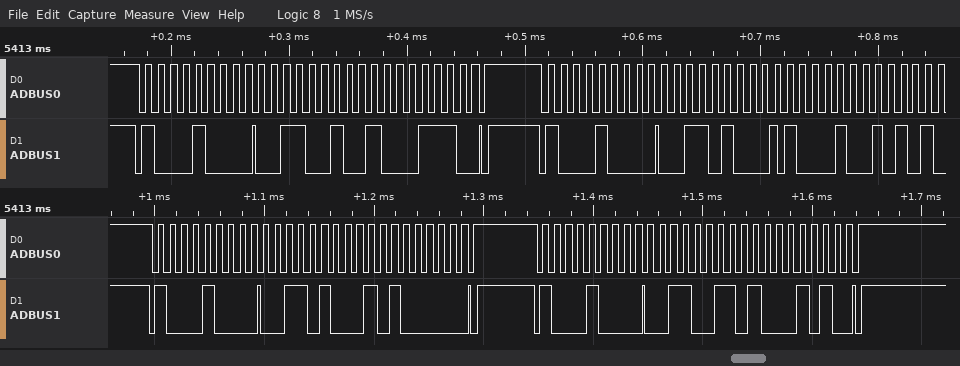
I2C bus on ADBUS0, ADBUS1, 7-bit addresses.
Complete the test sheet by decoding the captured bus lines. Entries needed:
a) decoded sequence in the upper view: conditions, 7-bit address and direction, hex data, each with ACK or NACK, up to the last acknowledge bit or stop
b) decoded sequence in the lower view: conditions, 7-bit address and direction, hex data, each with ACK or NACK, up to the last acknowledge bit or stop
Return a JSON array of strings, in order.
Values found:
["start, address 44 write ACK, 32 ACK, 8E ACK, stop, start, address 44 write ACK, 34 ACK, repeated start, address 44 read ACK", "start, address 44 write ACK, 34 ACK, A0 ACK, stop, start, address 44 write ACK, 33 ACK, 8A ACK, stop"]
